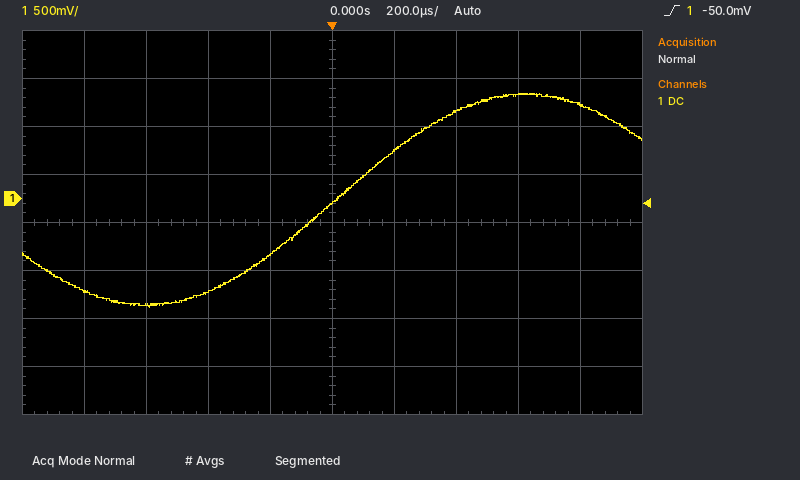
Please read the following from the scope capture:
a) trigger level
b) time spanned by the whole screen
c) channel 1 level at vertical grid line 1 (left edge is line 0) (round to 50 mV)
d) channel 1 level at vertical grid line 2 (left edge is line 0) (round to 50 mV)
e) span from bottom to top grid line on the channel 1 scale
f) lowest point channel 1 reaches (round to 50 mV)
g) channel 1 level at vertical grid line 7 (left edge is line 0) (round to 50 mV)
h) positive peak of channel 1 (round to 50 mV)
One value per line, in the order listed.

-50.0 mV
2 ms
-950 mV
-1.10 V
4 V
-1.15 V
900 mV
1.10 V
